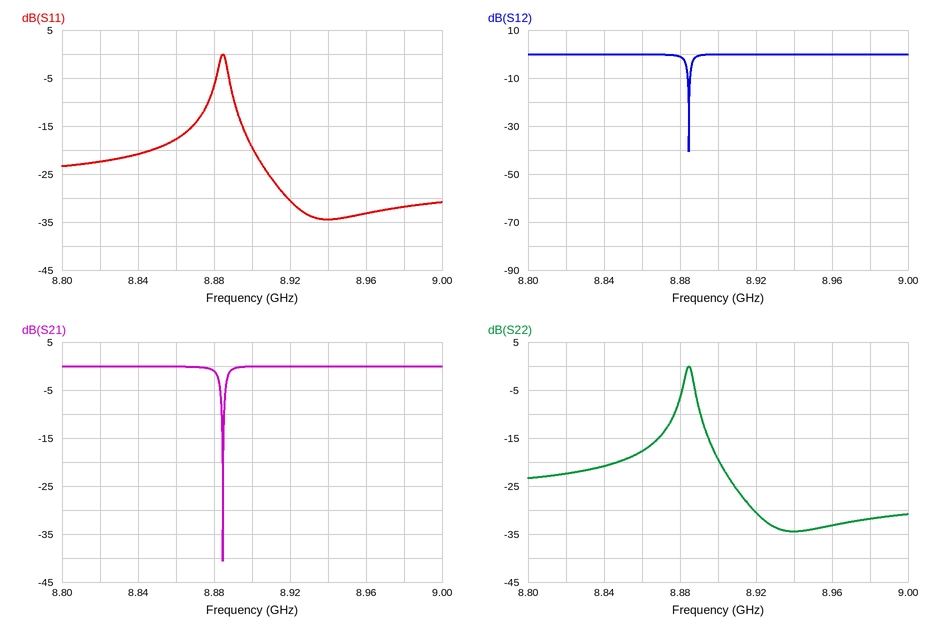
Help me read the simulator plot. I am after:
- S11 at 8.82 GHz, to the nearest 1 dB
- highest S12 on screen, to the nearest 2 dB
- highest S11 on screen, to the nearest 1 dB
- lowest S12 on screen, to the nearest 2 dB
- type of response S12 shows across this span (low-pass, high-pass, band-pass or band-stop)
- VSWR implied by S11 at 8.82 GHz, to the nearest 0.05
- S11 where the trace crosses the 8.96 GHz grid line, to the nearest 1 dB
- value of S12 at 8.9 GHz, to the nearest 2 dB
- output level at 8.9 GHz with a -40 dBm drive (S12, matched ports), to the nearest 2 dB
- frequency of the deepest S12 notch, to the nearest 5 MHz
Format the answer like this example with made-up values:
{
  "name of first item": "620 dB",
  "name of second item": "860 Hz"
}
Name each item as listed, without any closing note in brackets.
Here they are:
{
  "S11 at 8.82 GHz, to the nearest 1 dB": "-22 dB",
  "highest S12 on screen, to the nearest 2 dB": "0 dB",
  "highest S11 on screen, to the nearest 1 dB": "0 dB",
  "lowest S12 on screen, to the nearest 2 dB": "-40 dB",
  "type of response S12 shows across this span": "band-stop",
  "VSWR implied by S11 at 8.82 GHz, to the nearest 0.05": "1.15",
  "S11 where the trace crosses the 8.96 GHz grid line, to the nearest 1 dB": "-33 dB",
  "value of S12 at 8.9 GHz, to the nearest 2 dB": "0 dB",
  "output level at 8.9 GHz with a -40 dBm drive (S12, matched ports), to the nearest 2 dB": "-40 dBm",
  "frequency of the deepest S12 notch, to the nearest 5 MHz": "8.885 GHz"
}
